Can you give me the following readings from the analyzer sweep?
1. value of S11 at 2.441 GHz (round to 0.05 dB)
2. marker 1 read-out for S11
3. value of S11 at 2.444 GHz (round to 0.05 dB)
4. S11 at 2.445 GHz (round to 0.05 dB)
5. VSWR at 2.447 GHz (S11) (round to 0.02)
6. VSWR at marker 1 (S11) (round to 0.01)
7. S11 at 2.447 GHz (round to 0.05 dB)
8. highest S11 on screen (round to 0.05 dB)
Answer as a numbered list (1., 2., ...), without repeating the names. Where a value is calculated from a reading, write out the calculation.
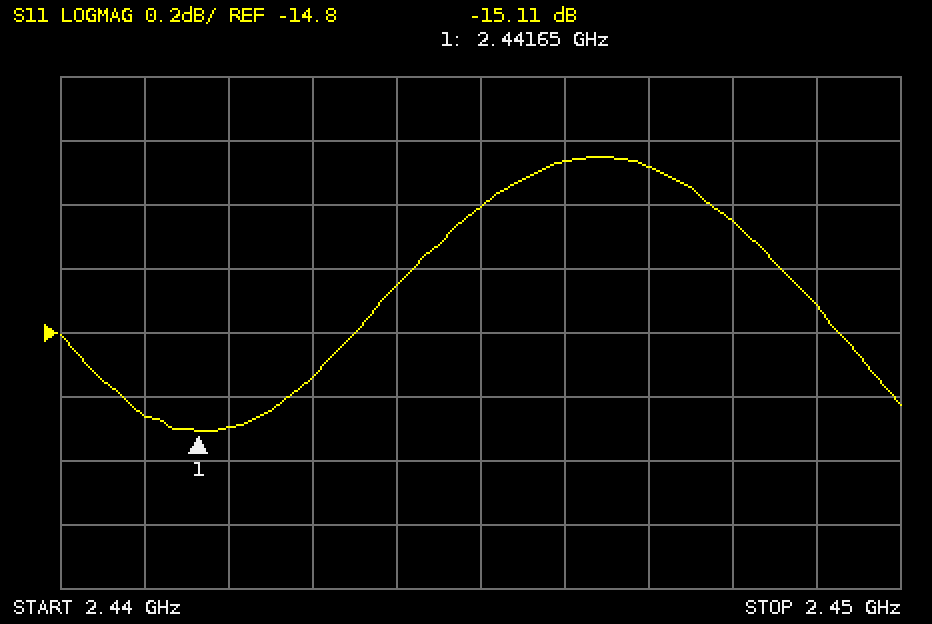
1. -15.05 dB
2. -15.11 dB
3. -14.65 dB
4. -14.40 dB
5. |Γ| = 10^(-14.3/20) = 0.1928; VSWR = (1 + 0.1928)/(1 − 0.1928) ≈ 1.48
6. (1 + 0.1756)/(1 − 0.1756) ≈ 1.43
7. -14.30 dB
8. -14.25 dB
